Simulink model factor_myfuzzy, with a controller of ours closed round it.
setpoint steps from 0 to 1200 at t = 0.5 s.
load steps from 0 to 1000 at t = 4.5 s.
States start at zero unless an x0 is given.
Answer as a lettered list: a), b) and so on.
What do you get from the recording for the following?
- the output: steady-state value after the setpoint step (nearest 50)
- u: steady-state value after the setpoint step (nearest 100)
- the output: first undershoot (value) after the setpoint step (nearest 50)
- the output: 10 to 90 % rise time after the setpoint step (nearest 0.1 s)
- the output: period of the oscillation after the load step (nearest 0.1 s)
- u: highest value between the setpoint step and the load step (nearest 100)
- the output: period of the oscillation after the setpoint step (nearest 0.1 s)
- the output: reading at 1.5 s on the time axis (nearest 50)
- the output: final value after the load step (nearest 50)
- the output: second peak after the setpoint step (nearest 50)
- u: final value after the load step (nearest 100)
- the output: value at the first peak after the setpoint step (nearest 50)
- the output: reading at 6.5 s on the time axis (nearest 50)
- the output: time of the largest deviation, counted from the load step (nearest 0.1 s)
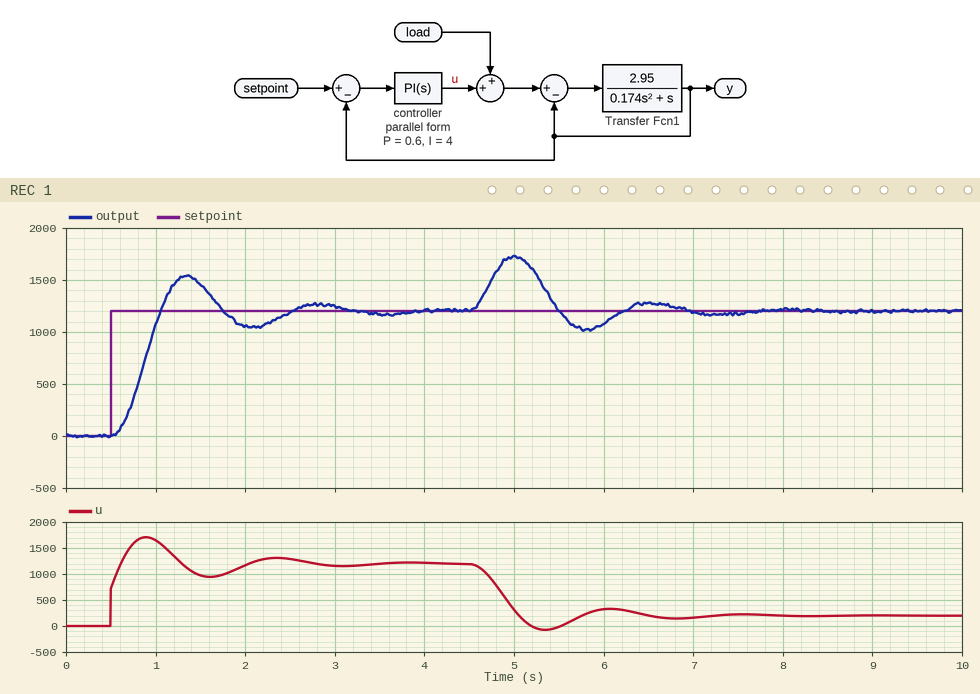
a) 1200
b) 1200
c) 1050
d) 0.4 s
e) 1.5 s
f) 1700
g) 1.5 s
h) 1450
i) 1200
j) 1250
k) 200
l) 1550
m) 1300
n) 0.5 s
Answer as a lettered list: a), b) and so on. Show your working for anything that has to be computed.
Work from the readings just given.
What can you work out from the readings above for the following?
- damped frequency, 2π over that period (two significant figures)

a) 2π / 1.5 = 4.2 rad/s
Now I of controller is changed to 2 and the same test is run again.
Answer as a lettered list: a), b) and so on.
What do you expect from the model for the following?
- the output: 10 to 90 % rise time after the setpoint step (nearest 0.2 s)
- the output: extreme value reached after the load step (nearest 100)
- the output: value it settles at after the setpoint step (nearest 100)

a) 0.6 s
b) 1800
c) 1200
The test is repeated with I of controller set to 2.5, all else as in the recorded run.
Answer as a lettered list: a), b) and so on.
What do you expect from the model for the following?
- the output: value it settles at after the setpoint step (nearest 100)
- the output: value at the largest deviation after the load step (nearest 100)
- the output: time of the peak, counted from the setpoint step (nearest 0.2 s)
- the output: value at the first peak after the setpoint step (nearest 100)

a) 1200
b) 1800
c) 1.0 s
d) 1300
